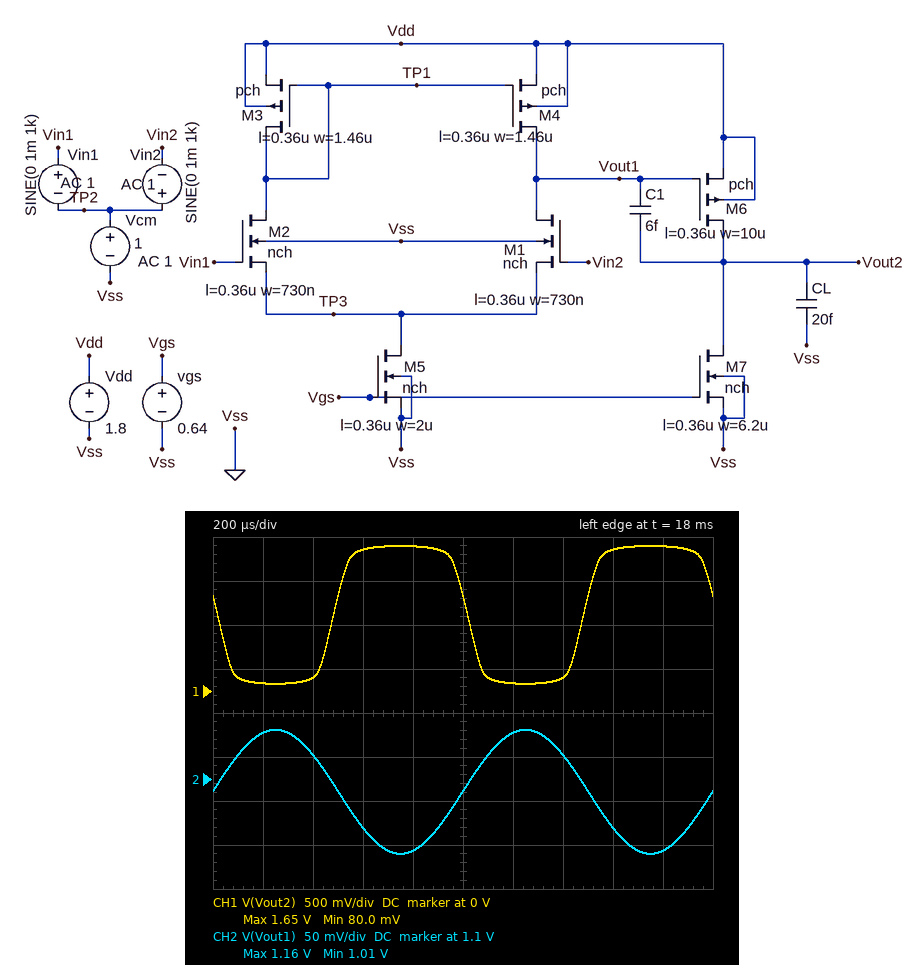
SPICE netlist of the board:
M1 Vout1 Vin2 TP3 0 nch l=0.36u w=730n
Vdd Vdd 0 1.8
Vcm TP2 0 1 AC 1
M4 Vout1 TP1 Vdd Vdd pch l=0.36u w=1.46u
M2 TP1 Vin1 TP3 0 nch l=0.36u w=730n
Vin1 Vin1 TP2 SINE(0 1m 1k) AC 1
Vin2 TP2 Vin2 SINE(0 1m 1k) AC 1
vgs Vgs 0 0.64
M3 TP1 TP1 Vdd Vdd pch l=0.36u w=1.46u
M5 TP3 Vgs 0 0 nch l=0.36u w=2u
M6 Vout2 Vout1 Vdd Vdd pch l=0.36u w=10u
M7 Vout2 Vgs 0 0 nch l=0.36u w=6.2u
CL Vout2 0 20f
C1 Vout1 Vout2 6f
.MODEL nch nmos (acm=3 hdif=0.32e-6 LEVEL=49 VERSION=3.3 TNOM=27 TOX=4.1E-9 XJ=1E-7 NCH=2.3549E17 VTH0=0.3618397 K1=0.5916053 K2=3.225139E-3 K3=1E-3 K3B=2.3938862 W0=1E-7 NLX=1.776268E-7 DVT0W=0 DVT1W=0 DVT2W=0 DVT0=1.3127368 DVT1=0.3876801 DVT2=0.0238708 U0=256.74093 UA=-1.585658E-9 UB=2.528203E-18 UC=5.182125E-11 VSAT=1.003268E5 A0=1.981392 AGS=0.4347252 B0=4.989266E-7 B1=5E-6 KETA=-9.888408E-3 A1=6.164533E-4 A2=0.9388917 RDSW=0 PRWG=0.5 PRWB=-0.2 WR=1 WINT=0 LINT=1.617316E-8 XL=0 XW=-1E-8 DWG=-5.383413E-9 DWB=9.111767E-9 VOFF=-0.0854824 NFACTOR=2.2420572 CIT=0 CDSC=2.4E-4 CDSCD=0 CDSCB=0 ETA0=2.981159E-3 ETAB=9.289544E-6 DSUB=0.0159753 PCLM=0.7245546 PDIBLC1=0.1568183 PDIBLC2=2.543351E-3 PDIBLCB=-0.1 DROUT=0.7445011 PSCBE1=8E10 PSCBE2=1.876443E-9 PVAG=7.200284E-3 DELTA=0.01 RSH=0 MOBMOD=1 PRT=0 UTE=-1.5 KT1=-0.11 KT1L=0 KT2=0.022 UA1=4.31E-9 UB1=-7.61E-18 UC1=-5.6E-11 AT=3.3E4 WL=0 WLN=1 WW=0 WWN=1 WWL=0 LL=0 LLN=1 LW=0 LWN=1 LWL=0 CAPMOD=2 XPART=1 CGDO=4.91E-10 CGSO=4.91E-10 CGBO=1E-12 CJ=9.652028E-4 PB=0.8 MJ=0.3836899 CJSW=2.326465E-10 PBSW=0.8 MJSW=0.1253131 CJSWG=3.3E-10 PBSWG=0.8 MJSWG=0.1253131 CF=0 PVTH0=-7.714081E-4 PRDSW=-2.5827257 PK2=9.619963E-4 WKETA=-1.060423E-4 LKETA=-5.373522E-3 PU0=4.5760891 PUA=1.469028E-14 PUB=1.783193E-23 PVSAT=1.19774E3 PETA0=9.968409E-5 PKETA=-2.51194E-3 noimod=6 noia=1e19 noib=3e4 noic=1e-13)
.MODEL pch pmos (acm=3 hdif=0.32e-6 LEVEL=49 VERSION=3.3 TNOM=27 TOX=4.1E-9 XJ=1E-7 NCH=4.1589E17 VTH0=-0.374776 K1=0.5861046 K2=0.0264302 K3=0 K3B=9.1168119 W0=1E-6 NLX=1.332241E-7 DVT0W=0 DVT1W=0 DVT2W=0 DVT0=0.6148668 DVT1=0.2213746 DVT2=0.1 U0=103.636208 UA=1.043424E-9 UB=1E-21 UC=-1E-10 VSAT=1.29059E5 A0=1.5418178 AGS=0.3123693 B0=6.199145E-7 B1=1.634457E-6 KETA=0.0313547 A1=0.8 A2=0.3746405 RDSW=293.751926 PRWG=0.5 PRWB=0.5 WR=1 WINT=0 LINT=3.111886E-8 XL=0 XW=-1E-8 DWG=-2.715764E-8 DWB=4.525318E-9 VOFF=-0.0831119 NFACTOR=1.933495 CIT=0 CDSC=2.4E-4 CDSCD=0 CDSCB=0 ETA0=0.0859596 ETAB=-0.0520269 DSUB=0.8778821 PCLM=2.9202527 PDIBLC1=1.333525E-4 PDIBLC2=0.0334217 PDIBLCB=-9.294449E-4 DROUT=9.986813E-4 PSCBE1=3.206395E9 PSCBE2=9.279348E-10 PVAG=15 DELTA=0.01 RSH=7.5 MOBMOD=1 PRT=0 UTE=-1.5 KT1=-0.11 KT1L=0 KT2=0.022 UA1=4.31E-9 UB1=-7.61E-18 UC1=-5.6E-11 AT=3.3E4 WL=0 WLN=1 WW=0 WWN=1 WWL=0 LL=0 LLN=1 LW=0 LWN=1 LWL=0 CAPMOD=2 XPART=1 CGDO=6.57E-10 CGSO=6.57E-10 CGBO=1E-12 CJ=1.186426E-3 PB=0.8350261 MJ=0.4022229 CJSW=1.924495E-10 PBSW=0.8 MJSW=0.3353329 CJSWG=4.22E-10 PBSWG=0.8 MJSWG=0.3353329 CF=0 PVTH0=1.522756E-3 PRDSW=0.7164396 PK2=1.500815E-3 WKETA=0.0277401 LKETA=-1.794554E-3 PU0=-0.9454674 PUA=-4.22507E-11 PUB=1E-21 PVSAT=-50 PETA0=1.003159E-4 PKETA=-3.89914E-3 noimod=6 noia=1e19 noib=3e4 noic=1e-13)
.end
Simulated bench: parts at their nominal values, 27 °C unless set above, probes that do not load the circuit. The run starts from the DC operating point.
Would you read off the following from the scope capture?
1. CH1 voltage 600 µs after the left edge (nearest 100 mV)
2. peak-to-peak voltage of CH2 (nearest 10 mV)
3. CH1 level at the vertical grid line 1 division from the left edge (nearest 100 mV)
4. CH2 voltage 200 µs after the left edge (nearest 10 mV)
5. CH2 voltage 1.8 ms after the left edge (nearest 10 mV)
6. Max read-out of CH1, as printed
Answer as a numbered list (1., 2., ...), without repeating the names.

1. 1.6 V
2. 140 mV
3. 100 mV
4. 1.15 V
5. 1.02 V
6. 1.65 V
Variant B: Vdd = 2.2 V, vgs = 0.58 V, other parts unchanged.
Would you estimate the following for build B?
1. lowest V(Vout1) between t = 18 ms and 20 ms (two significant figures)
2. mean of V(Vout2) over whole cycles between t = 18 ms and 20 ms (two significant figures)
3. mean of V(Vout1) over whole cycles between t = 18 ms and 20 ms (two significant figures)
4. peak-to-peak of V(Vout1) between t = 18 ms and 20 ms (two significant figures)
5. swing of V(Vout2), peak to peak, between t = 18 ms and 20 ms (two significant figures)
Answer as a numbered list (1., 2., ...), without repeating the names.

1. 1.5 V
2. 1.1 V
3. 1.6 V
4. 160 mV
5. 2.1 V
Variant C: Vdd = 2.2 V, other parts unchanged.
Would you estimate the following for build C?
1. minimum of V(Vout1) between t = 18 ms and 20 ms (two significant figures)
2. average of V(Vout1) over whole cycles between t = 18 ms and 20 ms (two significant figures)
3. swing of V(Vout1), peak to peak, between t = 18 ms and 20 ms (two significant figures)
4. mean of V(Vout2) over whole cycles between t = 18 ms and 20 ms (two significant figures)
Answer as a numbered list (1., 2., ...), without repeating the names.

1. 1.4 V
2. 1.5 V
3. 150 mV
4. 1.1 V
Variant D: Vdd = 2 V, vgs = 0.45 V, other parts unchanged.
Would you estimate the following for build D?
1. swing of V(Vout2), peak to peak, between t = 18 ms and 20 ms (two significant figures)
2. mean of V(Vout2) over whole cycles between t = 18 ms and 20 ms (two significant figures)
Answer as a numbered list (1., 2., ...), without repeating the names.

1. 2.0 V
2. 1.0 V
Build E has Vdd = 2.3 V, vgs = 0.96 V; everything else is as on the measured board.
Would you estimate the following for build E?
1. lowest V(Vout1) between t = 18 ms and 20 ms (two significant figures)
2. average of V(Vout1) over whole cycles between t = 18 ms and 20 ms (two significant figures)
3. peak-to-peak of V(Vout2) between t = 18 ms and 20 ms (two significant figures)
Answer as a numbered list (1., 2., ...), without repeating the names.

1. 1.2 V
2. 1.3 V
3. 78 mV
